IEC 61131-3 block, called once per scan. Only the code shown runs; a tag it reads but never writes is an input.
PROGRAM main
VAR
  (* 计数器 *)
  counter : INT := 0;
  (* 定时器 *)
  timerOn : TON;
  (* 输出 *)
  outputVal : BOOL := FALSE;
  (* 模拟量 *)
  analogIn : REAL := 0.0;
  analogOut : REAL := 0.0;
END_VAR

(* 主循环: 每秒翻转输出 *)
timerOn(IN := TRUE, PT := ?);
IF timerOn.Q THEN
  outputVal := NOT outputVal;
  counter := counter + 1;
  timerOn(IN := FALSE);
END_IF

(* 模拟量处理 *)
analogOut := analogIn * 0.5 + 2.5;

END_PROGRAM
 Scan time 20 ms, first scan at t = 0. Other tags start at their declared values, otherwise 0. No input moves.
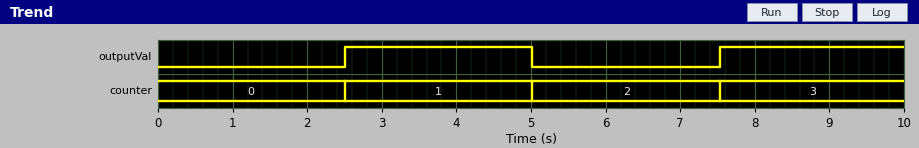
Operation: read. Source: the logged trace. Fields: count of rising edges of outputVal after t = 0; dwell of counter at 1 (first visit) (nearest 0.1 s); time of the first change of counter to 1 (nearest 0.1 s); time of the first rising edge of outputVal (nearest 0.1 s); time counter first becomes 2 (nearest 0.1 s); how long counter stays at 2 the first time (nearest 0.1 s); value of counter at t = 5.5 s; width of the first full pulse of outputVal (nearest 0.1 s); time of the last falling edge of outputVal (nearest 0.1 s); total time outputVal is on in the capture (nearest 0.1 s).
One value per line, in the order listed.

2
2.5 s
2.5 s
2.5 s
5.0 s
2.5 s
2
2.5 s
5.0 s
5.0 s
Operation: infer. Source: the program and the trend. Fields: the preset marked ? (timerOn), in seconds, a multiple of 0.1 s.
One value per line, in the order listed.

2.5 s
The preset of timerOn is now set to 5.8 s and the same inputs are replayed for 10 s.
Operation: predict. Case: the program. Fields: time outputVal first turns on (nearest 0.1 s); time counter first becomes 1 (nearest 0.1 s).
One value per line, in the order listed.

5.8 s
5.8 s
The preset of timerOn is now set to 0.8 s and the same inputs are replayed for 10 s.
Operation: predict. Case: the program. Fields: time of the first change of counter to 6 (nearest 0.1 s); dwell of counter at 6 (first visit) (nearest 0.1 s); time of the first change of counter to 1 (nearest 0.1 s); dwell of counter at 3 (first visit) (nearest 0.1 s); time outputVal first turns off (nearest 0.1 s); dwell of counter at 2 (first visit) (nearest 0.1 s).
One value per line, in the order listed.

4.9 s
0.8 s
0.8 s
0.8 s
1.6 s
0.8 s
